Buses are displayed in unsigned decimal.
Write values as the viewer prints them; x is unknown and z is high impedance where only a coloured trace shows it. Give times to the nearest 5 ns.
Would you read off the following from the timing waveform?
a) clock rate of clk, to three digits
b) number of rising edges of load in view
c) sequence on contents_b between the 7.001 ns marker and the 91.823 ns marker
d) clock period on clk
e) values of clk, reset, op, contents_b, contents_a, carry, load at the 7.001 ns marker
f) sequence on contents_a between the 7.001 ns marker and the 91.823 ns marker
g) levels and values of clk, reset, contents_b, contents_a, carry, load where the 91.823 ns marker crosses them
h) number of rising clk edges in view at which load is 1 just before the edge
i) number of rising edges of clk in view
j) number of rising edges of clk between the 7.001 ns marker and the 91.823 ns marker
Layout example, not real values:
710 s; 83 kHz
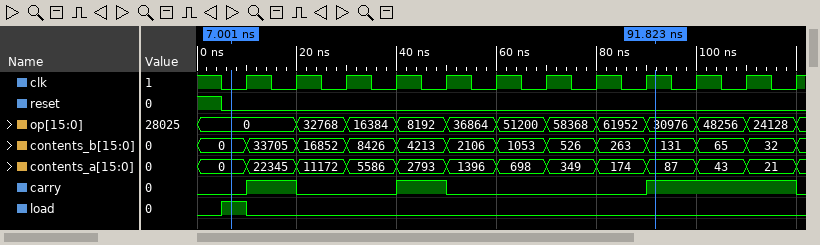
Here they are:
100 MHz; 1; 0, 33705, 16852, 8426, 4213, 2106, 1053, 526, 263, 131; 10 ns; clk=0, reset=0, op=0, contents_b=0, contents_a=0, carry=0, load=1; 0, 22345, 11172, 5586, 2793, 1396, 698, 349, 174, 87; clk=1, reset=0, contents_b=131, contents_a=87, carry=1, load=0; 1; 12; 9
